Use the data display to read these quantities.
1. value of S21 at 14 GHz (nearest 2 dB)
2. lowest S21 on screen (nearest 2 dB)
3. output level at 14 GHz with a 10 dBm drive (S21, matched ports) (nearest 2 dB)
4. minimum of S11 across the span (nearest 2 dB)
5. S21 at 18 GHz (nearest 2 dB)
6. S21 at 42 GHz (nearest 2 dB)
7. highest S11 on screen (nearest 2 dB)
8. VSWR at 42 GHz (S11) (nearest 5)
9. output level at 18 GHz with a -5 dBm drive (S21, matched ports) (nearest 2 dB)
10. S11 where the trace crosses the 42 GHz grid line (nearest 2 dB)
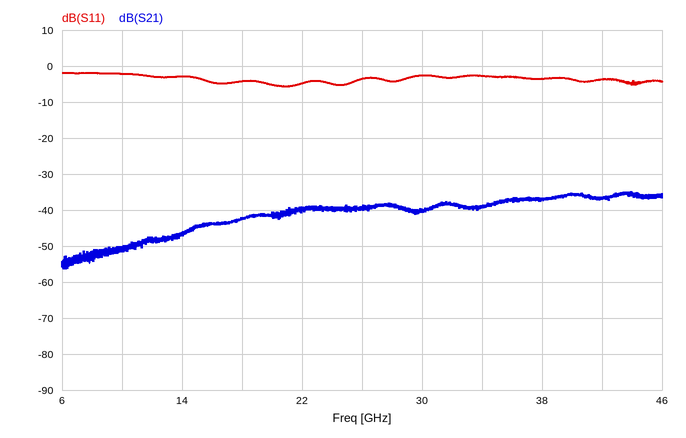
-46 dB
-56 dB
-36 dBm
-6 dB
-42 dB
-36 dB
-2 dB
5
-48 dBm
-4 dB
